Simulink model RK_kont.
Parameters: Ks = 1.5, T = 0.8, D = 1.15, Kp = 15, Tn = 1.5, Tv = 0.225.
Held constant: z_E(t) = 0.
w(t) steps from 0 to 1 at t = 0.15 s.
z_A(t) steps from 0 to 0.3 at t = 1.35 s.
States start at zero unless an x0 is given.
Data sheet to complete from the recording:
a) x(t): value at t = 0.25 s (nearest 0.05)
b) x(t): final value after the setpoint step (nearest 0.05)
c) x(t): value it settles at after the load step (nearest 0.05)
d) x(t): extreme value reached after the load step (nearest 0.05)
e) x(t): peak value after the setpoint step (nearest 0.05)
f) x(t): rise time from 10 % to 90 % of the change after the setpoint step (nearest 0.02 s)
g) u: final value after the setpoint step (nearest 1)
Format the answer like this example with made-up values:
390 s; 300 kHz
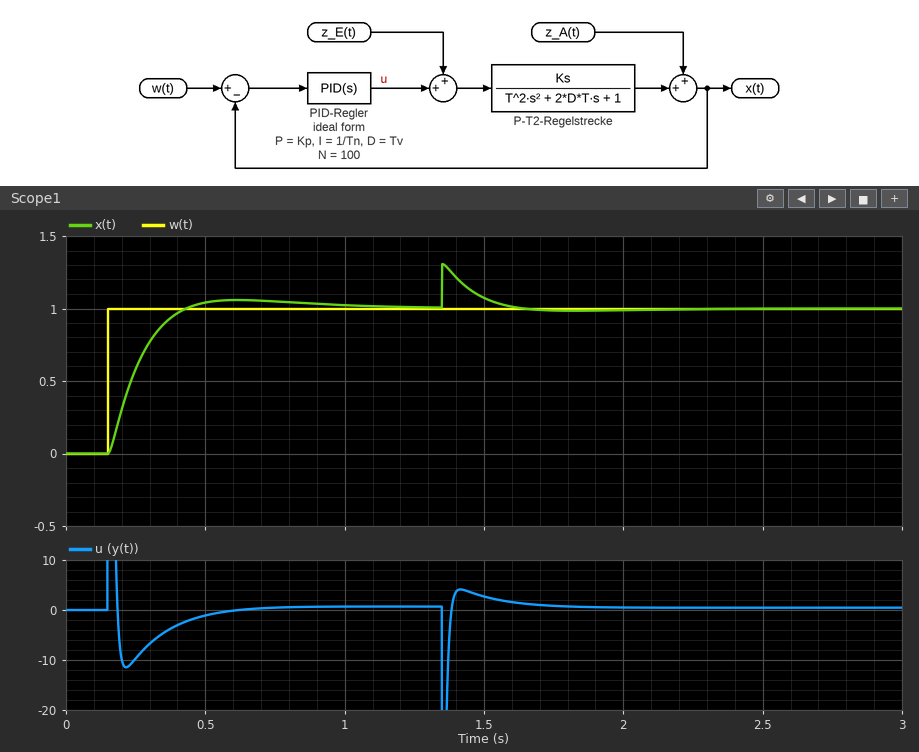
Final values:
0.60; 1.00; 1.00; 1.30; 1.05; 0.18 s; 1
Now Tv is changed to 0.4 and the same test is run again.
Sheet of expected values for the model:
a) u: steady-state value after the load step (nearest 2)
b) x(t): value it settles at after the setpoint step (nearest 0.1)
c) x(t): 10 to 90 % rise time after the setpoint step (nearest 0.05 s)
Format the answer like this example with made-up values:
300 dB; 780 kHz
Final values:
0; 1.0; 0.15 s
